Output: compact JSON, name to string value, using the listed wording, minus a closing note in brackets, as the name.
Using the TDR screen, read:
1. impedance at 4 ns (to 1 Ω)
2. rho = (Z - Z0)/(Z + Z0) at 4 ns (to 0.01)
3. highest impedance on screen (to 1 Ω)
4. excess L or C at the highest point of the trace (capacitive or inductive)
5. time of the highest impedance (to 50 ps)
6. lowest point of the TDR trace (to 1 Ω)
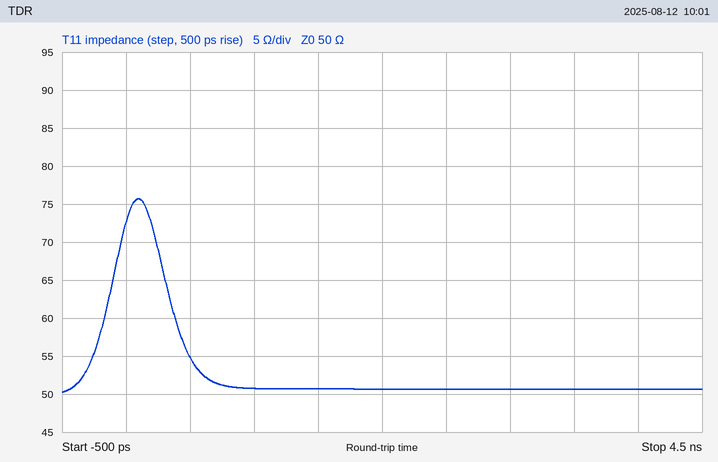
{"impedance at 4 ns": "51 Ω", "rho = (Z - Z0)/(Z + Z0) at 4 ns": "+0.01", "highest impedance on screen": "76 Ω", "excess L or C at the highest point of the trace": "inductive", "time of the highest impedance": "100 ps", "lowest point of the TDR trace": "50 Ω"}
